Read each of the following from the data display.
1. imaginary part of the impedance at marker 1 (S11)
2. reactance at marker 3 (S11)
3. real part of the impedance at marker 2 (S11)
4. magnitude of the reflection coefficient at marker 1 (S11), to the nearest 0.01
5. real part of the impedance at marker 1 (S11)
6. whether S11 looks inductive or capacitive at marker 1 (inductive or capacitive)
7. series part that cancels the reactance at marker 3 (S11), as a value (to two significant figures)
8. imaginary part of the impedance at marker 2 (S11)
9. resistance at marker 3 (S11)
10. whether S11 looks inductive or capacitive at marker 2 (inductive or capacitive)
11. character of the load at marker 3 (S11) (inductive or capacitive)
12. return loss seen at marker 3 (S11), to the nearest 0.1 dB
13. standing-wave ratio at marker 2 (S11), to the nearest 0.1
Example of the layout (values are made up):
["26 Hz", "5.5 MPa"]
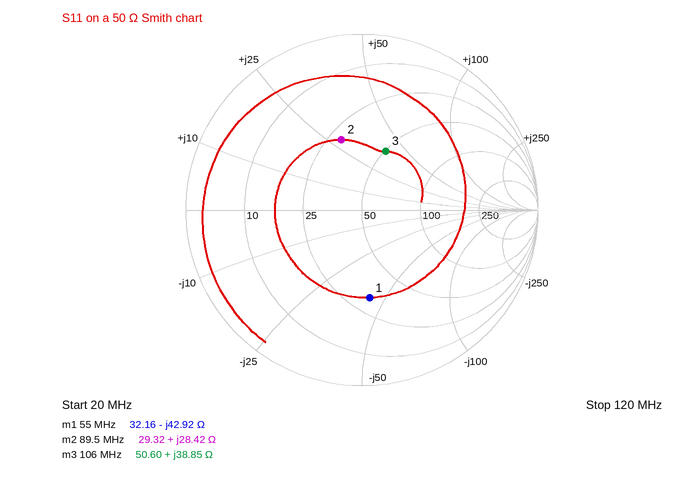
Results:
["-42.92 Ω", "+38.85 Ω", "29.32 Ω", "0.50", "32.16 Ω", "capacitive", "39 pF", "+28.42 Ω", "50.60 Ω", "inductive", "inductive", "8.9 dB", "2.4"]
